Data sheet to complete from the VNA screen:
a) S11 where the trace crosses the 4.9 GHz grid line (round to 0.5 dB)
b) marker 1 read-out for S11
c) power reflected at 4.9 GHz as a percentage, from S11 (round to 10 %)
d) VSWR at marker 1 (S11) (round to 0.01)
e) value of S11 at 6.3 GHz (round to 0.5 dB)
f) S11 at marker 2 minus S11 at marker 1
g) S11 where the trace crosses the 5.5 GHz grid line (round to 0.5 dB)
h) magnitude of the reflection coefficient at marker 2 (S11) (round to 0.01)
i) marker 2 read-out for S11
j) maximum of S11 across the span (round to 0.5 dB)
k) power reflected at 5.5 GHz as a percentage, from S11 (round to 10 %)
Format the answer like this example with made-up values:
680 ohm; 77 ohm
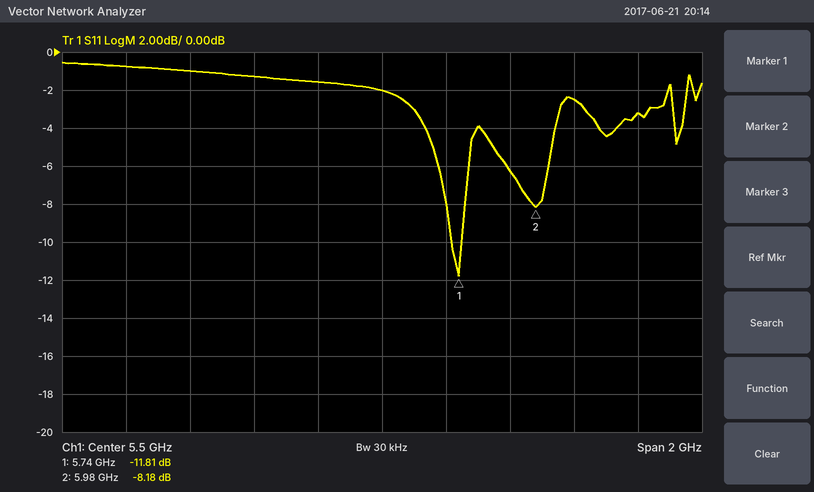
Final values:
-1.0 dB; -11.81 dB; 80 %; 1.69; -3.0 dB; 3.63 dB; -2.0 dB; 0.39; -8.18 dB; -0.5 dB; 60 %
